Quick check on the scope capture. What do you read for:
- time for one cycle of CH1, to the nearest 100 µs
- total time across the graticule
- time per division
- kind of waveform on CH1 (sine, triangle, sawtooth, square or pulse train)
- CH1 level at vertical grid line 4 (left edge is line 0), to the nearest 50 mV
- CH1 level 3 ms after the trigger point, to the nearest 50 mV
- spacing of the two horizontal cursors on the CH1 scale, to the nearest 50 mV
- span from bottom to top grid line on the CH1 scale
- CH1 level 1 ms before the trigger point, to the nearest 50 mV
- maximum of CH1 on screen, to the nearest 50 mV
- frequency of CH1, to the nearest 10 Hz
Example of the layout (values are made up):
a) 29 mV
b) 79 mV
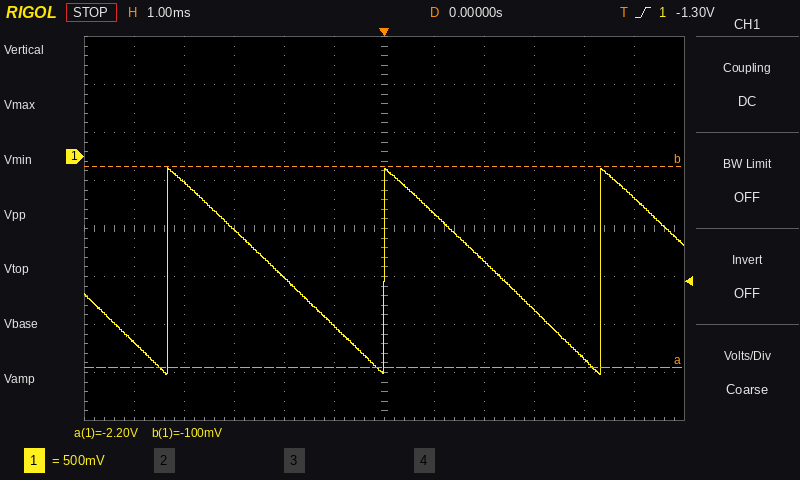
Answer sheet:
a) 4.3 ms
b) 12 ms
c) 1 ms
d) sawtooth
e) -1.25 V
f) -1.60 V
g) 2.10 V
h) 4 V
i) -1.75 V
j) -100 mV
k) 230 Hz
